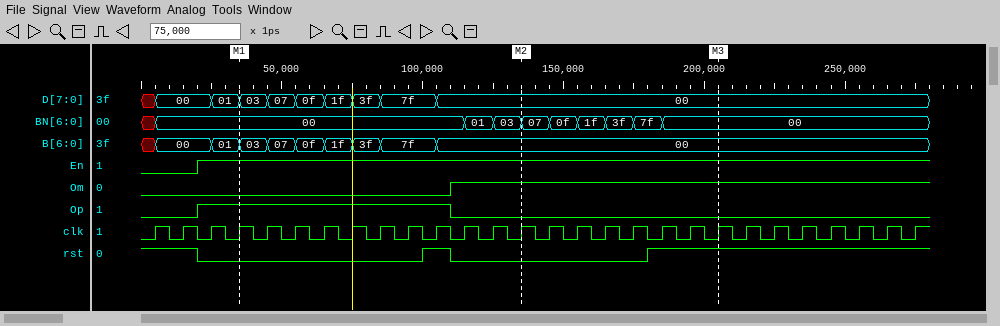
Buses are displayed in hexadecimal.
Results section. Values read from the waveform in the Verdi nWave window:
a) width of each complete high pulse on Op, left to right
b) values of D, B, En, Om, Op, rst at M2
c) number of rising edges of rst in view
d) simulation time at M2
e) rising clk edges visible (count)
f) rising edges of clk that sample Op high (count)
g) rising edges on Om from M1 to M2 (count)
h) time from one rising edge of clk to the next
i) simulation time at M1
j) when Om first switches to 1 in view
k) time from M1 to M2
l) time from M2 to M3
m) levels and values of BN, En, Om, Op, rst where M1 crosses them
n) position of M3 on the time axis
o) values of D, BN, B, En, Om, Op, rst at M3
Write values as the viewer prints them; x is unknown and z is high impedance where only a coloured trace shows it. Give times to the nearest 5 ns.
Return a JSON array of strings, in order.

["90 ns", "D=00, B=00, En=1, Om=1, Op=0, rst=0", "2", "135 ns", "28", "9", "1", "10 ns", "35 ns", "110 ns", "100 ns", "70 ns", "BN=00, En=1, Om=0, Op=1, rst=0", "205 ns", "D=00, BN=00, B=00, En=1, Om=1, Op=0, rst=1"]
